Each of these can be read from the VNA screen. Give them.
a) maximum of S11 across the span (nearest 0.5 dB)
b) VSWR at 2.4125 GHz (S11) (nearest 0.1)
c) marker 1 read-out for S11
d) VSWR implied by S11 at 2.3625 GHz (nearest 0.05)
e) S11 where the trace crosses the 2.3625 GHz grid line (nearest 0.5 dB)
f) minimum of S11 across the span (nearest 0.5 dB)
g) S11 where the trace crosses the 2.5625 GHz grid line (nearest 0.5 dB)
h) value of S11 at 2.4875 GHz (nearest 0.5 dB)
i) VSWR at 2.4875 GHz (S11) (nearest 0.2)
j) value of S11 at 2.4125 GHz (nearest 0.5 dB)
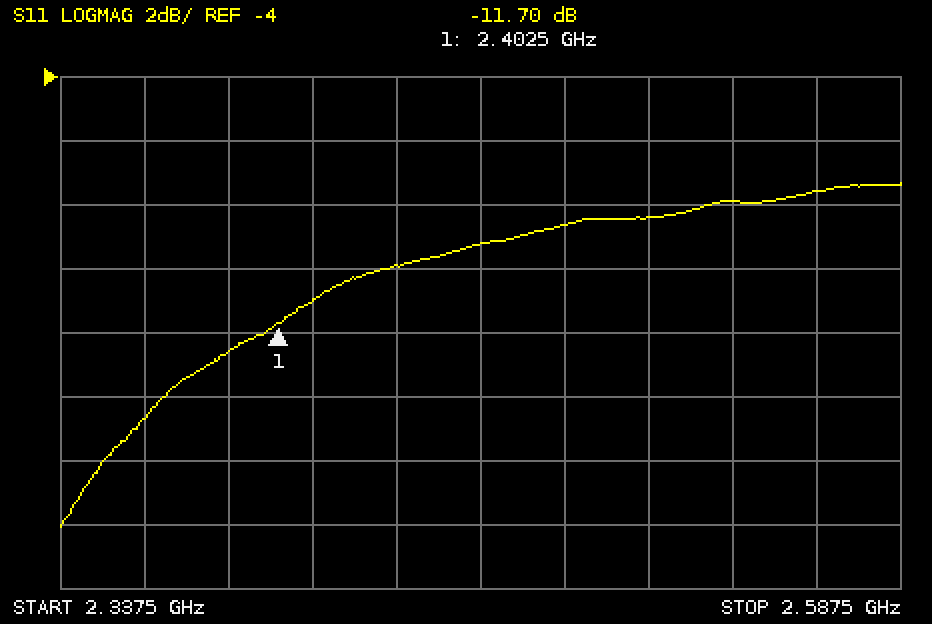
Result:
-7.5 dB
1.8
-11.70 dB
1.45
-14.5 dB
-18.0 dB
-7.5 dB
-8.5 dB
2.2
-11.0 dB
